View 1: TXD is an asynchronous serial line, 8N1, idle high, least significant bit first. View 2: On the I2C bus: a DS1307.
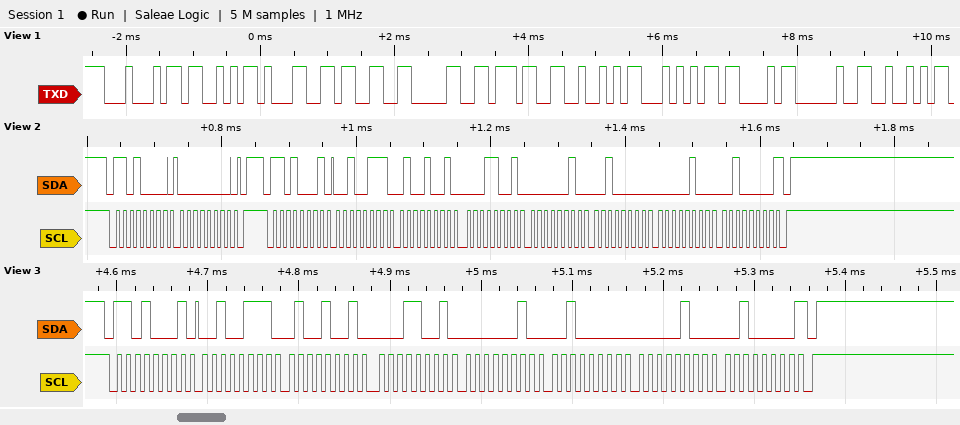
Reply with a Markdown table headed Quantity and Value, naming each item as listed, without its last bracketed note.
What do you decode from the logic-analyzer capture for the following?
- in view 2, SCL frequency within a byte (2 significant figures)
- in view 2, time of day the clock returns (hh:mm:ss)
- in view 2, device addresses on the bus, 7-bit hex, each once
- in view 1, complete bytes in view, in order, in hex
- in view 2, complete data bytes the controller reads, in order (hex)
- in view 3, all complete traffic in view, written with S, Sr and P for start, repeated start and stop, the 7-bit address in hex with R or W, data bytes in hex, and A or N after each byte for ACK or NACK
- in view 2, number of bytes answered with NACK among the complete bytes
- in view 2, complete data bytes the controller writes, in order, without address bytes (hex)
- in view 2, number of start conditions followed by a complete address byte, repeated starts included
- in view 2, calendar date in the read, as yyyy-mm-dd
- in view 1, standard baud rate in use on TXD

| Quantity | Value |
|---|---|
| in view 2, SCL frequency within a byte | 100 kHz |
| in view 2, time of day the clock returns | 19:49:27 |
| in view 2, device addresses on the bus, 7-bit hex, each once | 0x68 |
| in view 1, complete bytes in view, in order, in hex | 0x44 0x53 0x31 0x33 0x30 0x37 0x52 0x54 0x43 0x20 0x52 |
| in view 2, complete data bytes the controller reads, in order | 27 49 19 02 20 04 20 |
| in view 3, all complete traffic in view, written with S, Sr and P for start, repeated start and stop, the 7-bit address in hex with R or W, data bytes in hex, and A or N after each byte for ACK or NACK | S 68R A 27 A 49 A 19 A 02 A 20 A 04 A 20 N P |
| in view 2, number of bytes answered with NACK among the complete bytes | 1 |
| in view 2, complete data bytes the controller writes, in order, without address bytes | 00 |
| in view 2, number of start conditions followed by a complete address byte, repeated starts included | 2 |
| in view 2, calendar date in the read, as yyyy-mm-dd | 2020-04-20 |
| in view 1, standard baud rate in use on TXD | 9600 baud |
